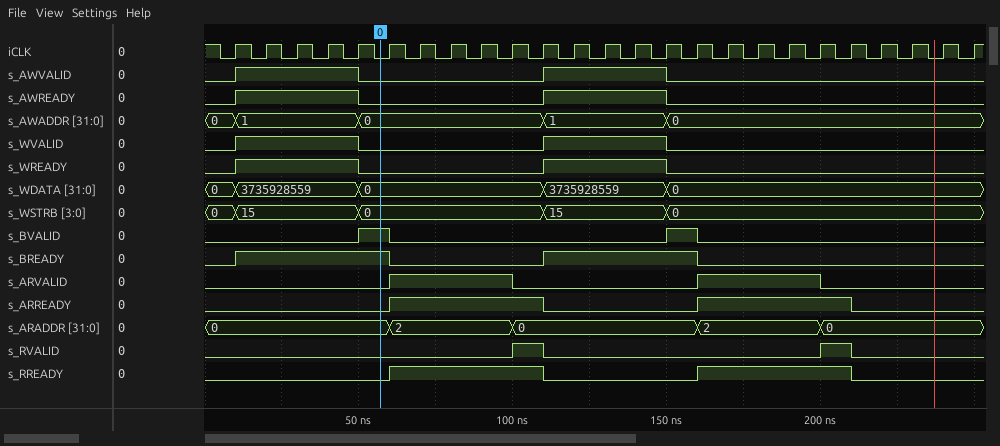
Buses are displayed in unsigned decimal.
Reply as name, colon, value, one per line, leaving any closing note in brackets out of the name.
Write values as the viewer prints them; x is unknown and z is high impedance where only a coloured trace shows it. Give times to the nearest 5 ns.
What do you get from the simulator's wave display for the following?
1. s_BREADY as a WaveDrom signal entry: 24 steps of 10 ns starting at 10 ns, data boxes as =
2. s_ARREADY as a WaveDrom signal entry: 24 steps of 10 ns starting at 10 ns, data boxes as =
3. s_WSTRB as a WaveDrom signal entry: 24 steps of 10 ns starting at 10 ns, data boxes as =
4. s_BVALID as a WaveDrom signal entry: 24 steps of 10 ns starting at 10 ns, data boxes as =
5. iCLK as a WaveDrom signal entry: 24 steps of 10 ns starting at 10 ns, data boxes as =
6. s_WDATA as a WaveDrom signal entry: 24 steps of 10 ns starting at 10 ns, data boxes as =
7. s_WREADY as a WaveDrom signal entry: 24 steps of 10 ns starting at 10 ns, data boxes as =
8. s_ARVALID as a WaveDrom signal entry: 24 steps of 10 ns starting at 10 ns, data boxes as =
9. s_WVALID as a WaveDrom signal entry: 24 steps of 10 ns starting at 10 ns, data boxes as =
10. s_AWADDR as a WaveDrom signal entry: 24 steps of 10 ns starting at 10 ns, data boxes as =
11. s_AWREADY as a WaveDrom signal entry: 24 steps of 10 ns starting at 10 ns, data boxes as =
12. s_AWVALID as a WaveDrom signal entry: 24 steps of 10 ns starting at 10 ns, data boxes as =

s_BREADY as a WaveDrom signal entry: 24 steps of 10 ns starting at 10 ns, data boxes as =: {name: 's_BREADY', wave: '1....0....1....0........'}
s_ARREADY as a WaveDrom signal entry: 24 steps of 10 ns starting at 10 ns, data boxes as =: {name: 's_ARREADY', wave: '0....1....0....1....0...'}
s_WSTRB as a WaveDrom signal entry: 24 steps of 10 ns starting at 10 ns, data boxes as =: {name: 's_WSTRB', wave: '=...=.....=...=.........', data: '15 0 15 0'}
s_BVALID as a WaveDrom signal entry: 24 steps of 10 ns starting at 10 ns, data boxes as =: {name: 's_BVALID', wave: '0...10........10........'}
iCLK as a WaveDrom signal entry: 24 steps of 10 ns starting at 10 ns, data boxes as =: {name: 'iCLK', wave: 'p.......................'}
s_WDATA as a WaveDrom signal entry: 24 steps of 10 ns starting at 10 ns, data boxes as =: {name: 's_WDATA', wave: '=...=.....=...=.........', data: '3735928559 0 3735928559 0'}
s_WREADY as a WaveDrom signal entry: 24 steps of 10 ns starting at 10 ns, data boxes as =: {name: 's_WREADY', wave: '1...0.....1...0.........'}
s_ARVALID as a WaveDrom signal entry: 24 steps of 10 ns starting at 10 ns, data boxes as =: {name: 's_ARVALID', wave: '0....1...0.....1...0....'}
s_WVALID as a WaveDrom signal entry: 24 steps of 10 ns starting at 10 ns, data boxes as =: {name: 's_WVALID', wave: '1...0.....1...0.........'}
s_AWADDR as a WaveDrom signal entry: 24 steps of 10 ns starting at 10 ns, data boxes as =: {name: 's_AWADDR', wave: '=...=.....=...=.........', data: '1 0 1 0'}
s_AWREADY as a WaveDrom signal entry: 24 steps of 10 ns starting at 10 ns, data boxes as =: {name: 's_AWREADY', wave: '1...0.....1...0.........'}
s_AWVALID as a WaveDrom signal entry: 24 steps of 10 ns starting at 10 ns, data boxes as =: {name: 's_AWVALID', wave: '1...0.....1...0.........'}
